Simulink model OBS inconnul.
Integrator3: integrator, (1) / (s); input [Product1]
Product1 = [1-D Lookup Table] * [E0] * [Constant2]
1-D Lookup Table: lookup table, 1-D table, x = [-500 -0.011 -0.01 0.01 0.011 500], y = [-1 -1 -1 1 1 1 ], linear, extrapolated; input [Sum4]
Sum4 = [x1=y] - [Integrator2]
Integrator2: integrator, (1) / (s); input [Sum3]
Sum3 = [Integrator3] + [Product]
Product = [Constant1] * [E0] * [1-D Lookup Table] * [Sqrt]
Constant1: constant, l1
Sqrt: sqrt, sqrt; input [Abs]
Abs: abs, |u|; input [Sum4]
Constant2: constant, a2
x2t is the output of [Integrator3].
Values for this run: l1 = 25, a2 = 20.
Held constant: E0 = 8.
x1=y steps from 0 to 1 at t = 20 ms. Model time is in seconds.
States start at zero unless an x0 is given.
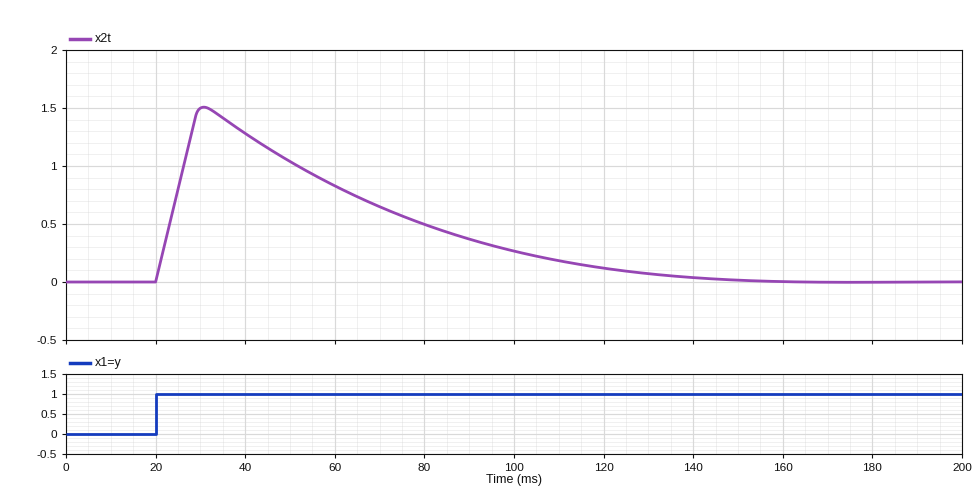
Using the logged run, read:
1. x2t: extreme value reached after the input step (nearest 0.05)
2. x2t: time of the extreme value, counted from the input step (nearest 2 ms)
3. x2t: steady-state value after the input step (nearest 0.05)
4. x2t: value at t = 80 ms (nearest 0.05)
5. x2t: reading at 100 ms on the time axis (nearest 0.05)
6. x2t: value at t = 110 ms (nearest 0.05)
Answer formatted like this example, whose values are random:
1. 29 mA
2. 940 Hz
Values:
1. 1.50
2. 10 ms
3. 0.00
4. 0.50
5. 0.25
6. 0.20
